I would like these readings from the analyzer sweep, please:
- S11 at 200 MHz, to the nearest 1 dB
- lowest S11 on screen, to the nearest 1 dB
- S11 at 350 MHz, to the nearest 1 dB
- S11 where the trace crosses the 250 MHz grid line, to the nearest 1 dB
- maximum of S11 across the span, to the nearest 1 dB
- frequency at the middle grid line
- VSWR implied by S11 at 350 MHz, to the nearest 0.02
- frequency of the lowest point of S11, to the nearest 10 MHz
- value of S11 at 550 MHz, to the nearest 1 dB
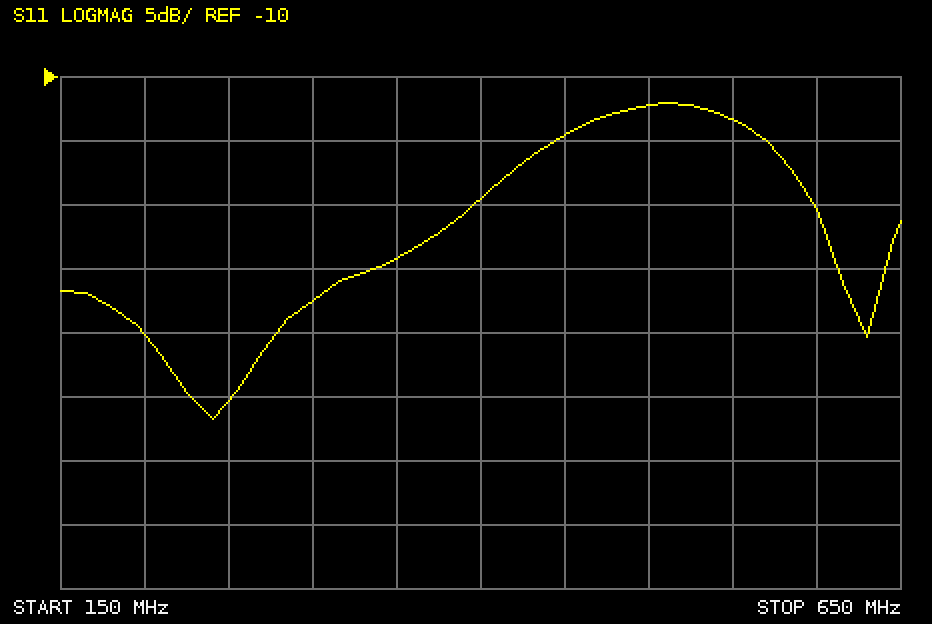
-30 dB
-37 dB
-24 dB
-35 dB
-12 dB
400 MHz
1.14
240 MHz
-13 dB
